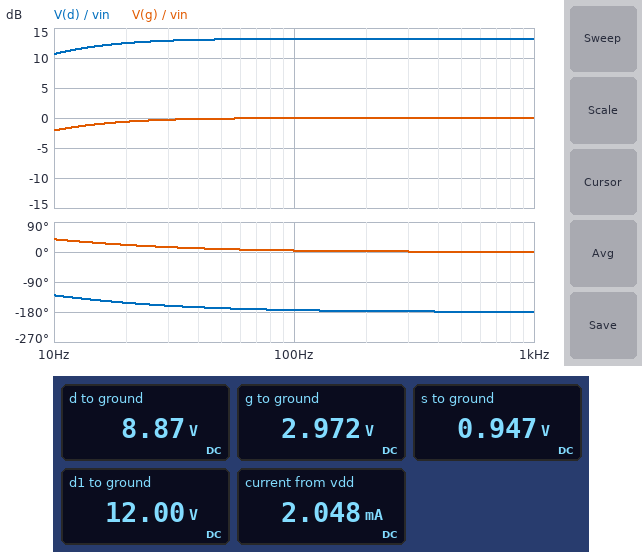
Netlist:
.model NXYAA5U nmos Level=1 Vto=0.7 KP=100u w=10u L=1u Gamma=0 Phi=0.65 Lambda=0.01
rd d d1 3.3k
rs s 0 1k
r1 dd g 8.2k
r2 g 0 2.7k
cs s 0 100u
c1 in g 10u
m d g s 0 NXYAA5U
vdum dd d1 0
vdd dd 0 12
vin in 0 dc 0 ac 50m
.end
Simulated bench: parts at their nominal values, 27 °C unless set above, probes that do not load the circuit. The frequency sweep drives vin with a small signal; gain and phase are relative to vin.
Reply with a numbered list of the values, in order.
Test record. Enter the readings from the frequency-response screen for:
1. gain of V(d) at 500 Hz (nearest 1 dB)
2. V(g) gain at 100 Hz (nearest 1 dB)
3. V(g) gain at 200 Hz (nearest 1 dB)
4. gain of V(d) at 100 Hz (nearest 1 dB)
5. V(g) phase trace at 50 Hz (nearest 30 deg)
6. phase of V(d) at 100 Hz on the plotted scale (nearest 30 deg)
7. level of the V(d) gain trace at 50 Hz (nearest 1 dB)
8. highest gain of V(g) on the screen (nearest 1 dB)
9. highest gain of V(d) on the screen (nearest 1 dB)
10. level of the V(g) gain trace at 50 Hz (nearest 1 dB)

1. 13 dB
2. 0 dB
3. 0 dB
4. 13 dB
5. 0 deg
6. -180 deg
7. 13 dB
8. 0 dB
9. 13 dB
10. 0 dB
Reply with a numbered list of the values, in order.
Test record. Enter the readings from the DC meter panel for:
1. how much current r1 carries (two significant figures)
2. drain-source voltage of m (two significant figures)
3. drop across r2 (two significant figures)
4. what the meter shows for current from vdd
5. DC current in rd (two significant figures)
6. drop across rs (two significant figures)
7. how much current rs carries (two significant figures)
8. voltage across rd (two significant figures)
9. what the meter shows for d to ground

1. 1.1 mA
2. 7.9 V
3. 3.0 V
4. 2.048 mA
5. 950 µA
6. 950 mV
7. 950 µA
8. 3.1 V
9. 8.87 V
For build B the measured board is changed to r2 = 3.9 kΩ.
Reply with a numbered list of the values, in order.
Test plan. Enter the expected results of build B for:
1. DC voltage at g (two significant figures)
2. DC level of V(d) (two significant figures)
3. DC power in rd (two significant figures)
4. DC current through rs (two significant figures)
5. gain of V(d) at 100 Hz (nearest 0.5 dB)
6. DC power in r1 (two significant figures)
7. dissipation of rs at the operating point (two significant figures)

1. 3.9 V
2. 7.1 V
3. 7.3 mW
4. 1.5 mA
5. 15.0 dB
6. 8.1 mW
7. 2.2 mW
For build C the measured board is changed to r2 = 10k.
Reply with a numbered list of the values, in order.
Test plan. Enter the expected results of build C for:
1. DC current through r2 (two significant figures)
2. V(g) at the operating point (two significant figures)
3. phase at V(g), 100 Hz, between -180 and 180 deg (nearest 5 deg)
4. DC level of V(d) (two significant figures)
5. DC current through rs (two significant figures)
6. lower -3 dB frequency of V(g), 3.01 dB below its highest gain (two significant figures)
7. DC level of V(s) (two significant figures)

1. 660 µA
2. 6.6 V
3. 0 deg
4. 3.5 V
5. 2.6 mA
6. 3.5 Hz
7. 2.6 V
